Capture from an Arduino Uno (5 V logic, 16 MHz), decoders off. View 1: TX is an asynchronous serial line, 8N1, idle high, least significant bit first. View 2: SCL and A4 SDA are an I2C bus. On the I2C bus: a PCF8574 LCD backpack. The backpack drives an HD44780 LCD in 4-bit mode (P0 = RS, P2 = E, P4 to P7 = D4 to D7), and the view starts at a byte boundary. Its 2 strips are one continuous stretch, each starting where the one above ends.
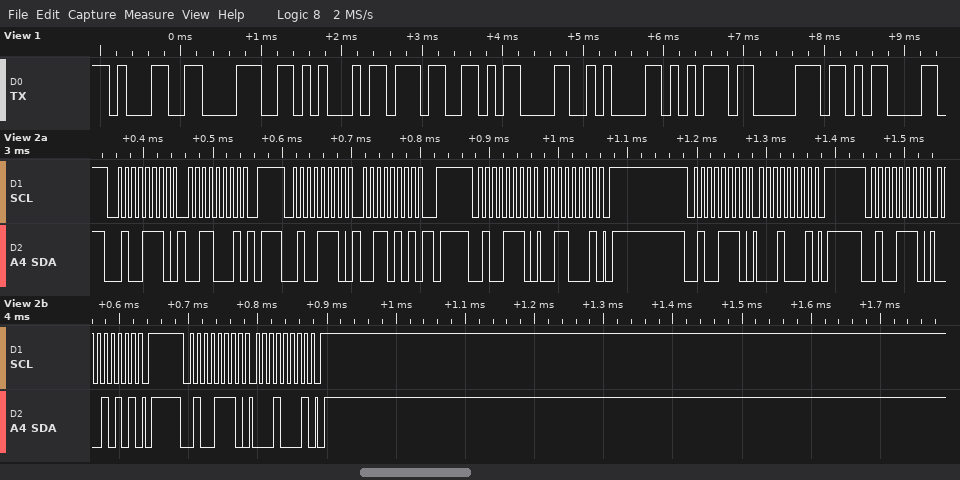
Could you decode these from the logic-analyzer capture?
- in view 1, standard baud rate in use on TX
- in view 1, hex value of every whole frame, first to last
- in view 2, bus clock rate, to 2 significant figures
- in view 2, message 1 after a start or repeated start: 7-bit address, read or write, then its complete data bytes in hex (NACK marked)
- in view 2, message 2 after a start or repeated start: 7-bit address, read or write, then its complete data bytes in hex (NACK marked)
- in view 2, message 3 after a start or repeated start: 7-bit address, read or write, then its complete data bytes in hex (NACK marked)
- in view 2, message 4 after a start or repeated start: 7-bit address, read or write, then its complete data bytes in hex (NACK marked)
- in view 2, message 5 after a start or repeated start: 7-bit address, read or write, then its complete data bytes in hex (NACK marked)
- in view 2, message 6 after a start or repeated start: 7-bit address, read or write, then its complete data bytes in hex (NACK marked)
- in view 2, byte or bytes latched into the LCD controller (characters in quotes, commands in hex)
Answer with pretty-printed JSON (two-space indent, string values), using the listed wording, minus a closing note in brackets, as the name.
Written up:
{
  "in view 1, standard baud rate in use on TX": "9600 baud",
  "in view 1, hex value of every whole frame, first to last": "31 38 45 37 0D 0A 75 70 0D",
  "in view 2, bus clock rate, to 2 significant figures": "100 kHz",
  "in view 2, message 1 after a start or repeated start: 7-bit address, read or write, then its complete data bytes in hex": "0x27 write: 31",
  "in view 2, message 2 after a start or repeated start: 7-bit address, read or write, then its complete data bytes in hex": "0x27 write: 35",
  "in view 2, message 3 after a start or repeated start: 7-bit address, read or write, then its complete data bytes in hex": "0x27 write: 31",
  "in view 2, message 4 after a start or repeated start: 7-bit address, read or write, then its complete data bytes in hex": "0x27 write: 11",
  "in view 2, message 5 after a start or repeated start: 7-bit address, read or write, then its complete data bytes in hex": "0x27 write: 15",
  "in view 2, message 6 after a start or repeated start: 7-bit address, read or write, then its complete data bytes in hex": "0x27 write: 11",
  "in view 2, byte or bytes latched into the LCD controller": "'1'"
}
